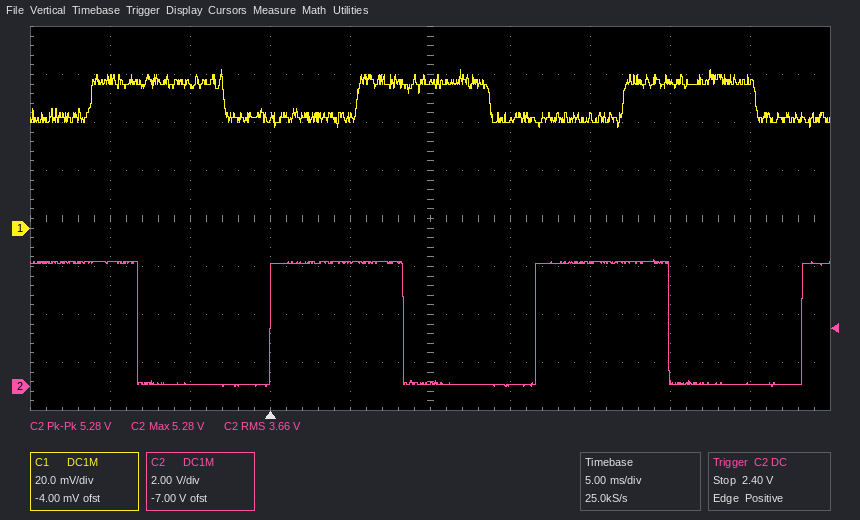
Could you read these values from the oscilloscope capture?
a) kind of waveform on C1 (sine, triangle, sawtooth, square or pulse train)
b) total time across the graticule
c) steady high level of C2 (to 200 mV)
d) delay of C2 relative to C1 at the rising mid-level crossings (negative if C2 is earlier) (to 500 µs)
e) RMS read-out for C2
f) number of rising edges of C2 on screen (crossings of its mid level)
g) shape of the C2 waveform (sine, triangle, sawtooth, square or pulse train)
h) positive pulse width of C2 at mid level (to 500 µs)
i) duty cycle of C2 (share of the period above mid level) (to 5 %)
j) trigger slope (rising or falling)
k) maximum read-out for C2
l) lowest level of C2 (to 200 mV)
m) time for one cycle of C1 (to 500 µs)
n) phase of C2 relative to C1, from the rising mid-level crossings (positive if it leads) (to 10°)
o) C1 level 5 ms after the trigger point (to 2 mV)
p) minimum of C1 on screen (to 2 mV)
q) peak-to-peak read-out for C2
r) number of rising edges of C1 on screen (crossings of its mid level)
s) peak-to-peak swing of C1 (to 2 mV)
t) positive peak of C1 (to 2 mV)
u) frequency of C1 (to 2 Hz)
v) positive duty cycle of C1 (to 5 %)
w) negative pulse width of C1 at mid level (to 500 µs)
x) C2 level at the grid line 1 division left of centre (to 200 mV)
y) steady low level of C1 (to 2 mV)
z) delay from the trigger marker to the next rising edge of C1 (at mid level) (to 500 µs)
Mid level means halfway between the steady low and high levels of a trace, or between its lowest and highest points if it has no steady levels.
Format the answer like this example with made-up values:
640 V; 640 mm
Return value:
square; 50 ms; 5.2 V; -5.5 ms; 3.66 V; 3; square; 8.5 ms; 50 %; rising; 5.28 V; 0.0 V; 16.5 ms; +120°; 46 mV; 42 mV; 5.28 V; 3; 24 mV; 66 mV; 60 Hz; 50 %; 8.5 ms; 5.2 V; 46 mV; 5.5 ms
